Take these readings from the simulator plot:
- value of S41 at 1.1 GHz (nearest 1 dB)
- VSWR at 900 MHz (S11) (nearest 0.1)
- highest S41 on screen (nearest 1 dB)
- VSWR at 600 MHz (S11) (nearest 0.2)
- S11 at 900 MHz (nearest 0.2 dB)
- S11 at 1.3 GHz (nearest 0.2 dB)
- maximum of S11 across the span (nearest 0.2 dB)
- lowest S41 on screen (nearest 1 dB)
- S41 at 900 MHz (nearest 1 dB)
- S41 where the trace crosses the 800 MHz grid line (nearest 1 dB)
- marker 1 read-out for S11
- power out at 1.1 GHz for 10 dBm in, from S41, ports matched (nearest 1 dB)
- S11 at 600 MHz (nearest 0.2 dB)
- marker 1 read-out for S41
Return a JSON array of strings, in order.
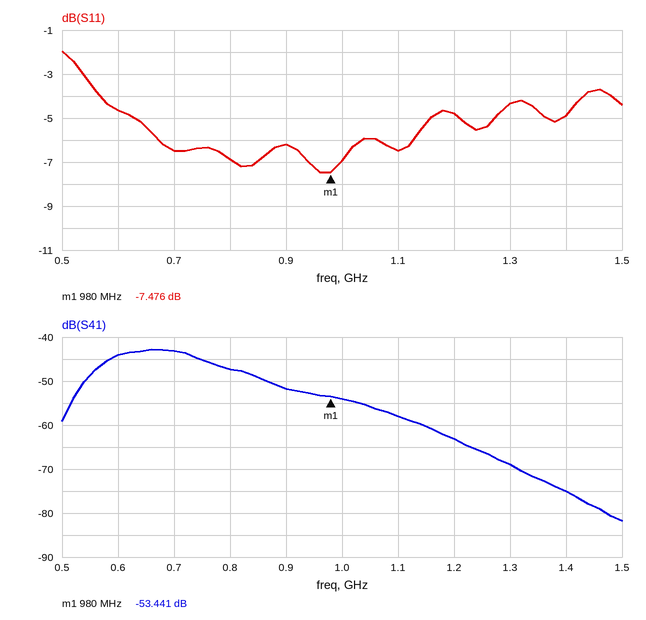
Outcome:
["-58 dB", "2.9", "-43 dB", "3.8", "-6.2 dB", "-4.4 dB", "-2.0 dB", "-82 dB", "-52 dB", "-47 dB", "-7.476 dB", "-48 dBm", "-4.6 dB", "-53.441 dB"]
